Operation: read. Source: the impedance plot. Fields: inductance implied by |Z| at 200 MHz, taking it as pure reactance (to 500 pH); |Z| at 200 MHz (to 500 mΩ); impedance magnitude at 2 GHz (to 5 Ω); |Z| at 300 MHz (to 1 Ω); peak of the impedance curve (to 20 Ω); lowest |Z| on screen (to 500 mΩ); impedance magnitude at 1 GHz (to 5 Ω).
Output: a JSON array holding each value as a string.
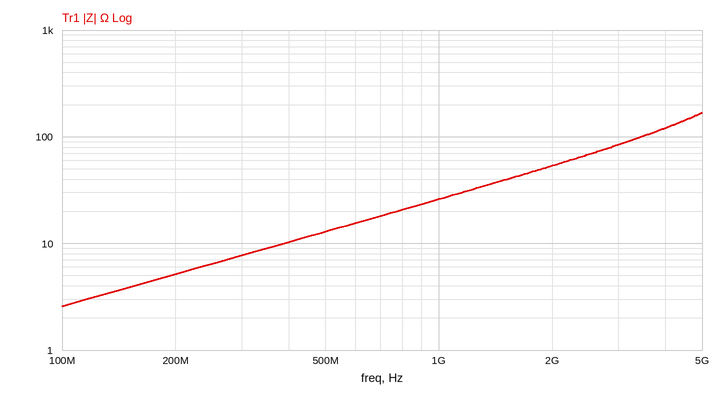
["4.0 nH", "5.0 Ω", "55 Ω", "8 Ω", "160 Ω", "2.5 Ω", "25 Ω"]
